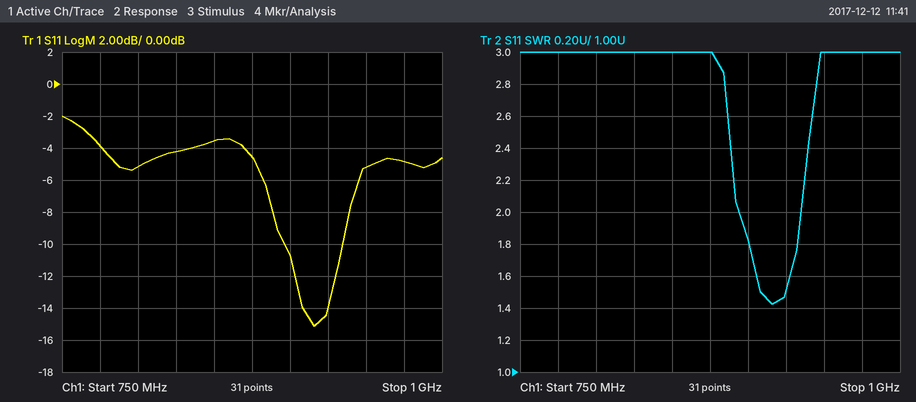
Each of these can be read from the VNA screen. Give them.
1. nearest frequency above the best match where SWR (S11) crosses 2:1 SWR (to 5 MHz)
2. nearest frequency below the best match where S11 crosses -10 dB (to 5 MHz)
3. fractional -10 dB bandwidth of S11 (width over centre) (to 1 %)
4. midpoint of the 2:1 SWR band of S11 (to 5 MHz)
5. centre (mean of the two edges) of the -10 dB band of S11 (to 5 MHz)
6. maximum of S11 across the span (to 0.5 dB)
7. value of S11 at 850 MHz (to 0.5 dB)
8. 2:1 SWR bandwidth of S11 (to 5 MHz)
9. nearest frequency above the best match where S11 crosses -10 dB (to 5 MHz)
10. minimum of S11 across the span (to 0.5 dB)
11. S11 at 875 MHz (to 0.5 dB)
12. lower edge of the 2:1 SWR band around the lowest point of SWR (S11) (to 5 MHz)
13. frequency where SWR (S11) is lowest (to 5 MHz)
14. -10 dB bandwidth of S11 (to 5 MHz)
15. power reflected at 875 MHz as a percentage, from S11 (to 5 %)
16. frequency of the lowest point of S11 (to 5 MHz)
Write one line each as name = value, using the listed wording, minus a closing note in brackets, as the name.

nearest frequency above the best match where SWR (S11) crosses 2:1 SWR = 935 MHz
nearest frequency below the best match where S11 crosses -10 dB = 895 MHz
fractional -10 dB bandwidth of S11 (width over centre) = 4 %
midpoint of the 2:1 SWR band of S11 = 915 MHz
centre (mean of the two edges) of the -10 dB band of S11 = 915 MHz
maximum of S11 across the span = -2.0 dB
value of S11 at 850 MHz = -3.5 dB
2:1 SWR bandwidth of S11 = 40 MHz
nearest frequency above the best match where S11 crosses -10 dB = 935 MHz
minimum of S11 across the span = -15.0 dB
S11 at 875 MHz = -4.5 dB
lower edge of the 2:1 SWR band around the lowest point of SWR (S11) = 895 MHz
frequency where SWR (S11) is lowest = 915 MHz
-10 dB bandwidth of S11 = 40 MHz
power reflected at 875 MHz as a percentage, from S11 = 35 %
frequency of the lowest point of S11 = 915 MHz
